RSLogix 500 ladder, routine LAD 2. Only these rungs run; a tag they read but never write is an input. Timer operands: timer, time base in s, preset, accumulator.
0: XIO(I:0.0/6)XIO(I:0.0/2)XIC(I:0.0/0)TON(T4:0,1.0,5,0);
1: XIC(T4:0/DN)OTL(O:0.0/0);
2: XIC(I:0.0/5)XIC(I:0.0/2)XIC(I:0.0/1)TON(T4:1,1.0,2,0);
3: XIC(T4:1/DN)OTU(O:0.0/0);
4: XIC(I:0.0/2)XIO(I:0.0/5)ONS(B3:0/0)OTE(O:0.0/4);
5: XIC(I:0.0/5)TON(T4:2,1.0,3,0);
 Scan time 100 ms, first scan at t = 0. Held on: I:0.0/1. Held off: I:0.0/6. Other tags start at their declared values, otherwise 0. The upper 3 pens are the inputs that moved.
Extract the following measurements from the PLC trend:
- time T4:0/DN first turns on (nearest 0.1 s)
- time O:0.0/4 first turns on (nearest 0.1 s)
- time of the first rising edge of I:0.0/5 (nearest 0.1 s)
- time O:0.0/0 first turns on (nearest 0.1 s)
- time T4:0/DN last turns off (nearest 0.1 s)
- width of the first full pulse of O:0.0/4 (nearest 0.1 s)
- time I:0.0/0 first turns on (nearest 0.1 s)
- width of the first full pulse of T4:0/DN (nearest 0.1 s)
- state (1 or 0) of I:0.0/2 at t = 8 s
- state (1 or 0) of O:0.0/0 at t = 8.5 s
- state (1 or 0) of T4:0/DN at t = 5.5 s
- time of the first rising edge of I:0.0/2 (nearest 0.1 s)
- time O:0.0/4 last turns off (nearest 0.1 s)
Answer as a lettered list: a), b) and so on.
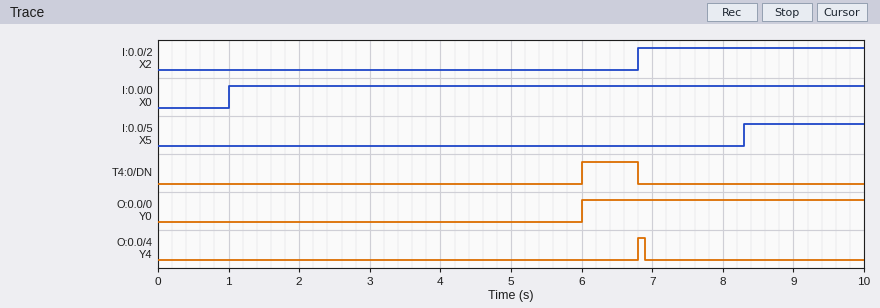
a) 6.0 s
b) 6.8 s
c) 8.3 s
d) 6.0 s
e) 6.8 s
f) 0.1 s
g) 1.0 s
h) 0.8 s
i) 1
j) 1
k) 0
l) 6.8 s
m) 6.9 s
